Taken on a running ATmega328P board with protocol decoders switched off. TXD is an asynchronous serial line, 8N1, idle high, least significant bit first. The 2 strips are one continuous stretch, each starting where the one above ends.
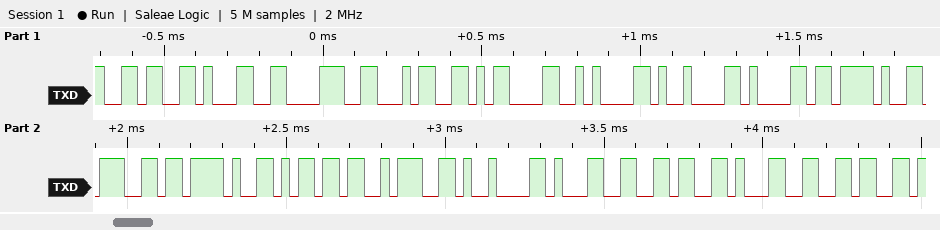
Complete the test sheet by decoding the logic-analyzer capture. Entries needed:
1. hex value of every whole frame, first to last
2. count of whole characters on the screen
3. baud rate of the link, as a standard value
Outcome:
36 31 38 34 0D 0A 09 61 2F 67 2F 6D 3A 09 31 36 31 36
18
38400 baud
